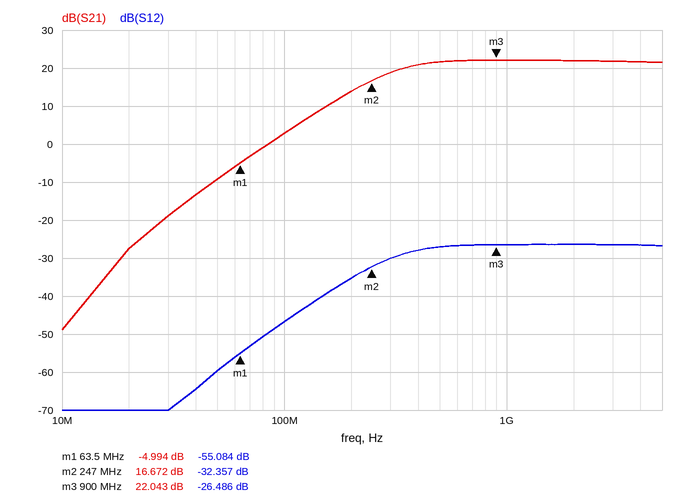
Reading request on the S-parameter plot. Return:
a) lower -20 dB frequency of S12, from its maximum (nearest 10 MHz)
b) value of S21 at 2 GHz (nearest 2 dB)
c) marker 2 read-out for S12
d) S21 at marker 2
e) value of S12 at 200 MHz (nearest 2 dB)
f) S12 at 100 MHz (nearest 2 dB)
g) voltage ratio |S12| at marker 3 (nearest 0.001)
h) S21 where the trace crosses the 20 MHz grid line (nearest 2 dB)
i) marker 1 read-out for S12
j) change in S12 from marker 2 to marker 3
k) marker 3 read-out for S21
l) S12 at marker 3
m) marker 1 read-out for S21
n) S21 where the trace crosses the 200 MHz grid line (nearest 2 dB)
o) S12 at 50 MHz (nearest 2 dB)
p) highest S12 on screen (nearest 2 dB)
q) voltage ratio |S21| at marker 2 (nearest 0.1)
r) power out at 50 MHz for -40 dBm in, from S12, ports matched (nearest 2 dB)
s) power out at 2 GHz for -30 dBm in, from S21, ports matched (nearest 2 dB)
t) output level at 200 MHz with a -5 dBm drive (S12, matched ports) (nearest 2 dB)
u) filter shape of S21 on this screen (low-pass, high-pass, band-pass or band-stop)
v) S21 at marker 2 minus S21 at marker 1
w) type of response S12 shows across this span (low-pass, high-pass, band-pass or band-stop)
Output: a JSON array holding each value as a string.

["100 MHz", "22 dB", "-32.357 dB", "16.672 dB", "-36 dB", "-46 dB", "0.047", "-28 dB", "-55.084 dB", "5.871 dB", "22.043 dB", "-26.486 dB", "-4.994 dB", "14 dB", "-60 dB", "-26 dB", "6.8", "-100 dBm", "-8 dBm", "-40 dBm", "high-pass", "21.666 dB", "high-pass"]
